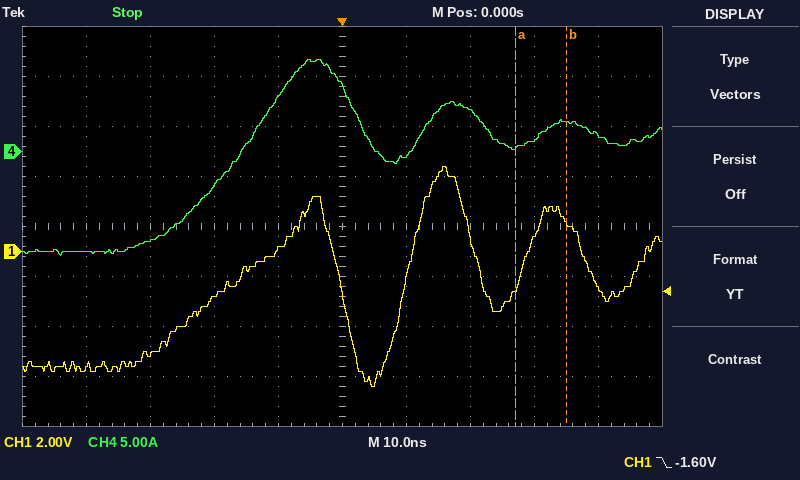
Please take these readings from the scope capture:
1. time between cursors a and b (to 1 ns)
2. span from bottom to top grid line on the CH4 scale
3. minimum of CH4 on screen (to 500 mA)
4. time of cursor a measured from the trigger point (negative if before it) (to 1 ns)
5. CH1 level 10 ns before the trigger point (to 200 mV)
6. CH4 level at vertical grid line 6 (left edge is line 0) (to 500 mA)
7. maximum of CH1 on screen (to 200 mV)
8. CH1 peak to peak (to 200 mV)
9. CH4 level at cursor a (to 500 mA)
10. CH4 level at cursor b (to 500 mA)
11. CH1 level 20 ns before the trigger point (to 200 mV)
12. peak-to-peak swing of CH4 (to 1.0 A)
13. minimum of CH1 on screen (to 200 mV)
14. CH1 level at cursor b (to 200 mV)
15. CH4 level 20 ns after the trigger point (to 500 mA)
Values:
8 ns
40 A
-10.5 A
+27 ns
0.0 V
-500 mA
3.4 V
8.8 V
500 mA
3.0 A
-1.8 V
20.0 A
-5.4 V
1.2 V
4.0 A
